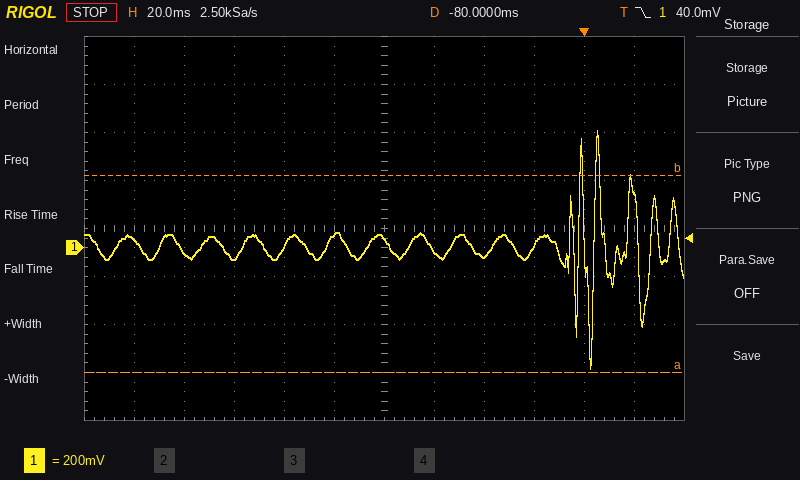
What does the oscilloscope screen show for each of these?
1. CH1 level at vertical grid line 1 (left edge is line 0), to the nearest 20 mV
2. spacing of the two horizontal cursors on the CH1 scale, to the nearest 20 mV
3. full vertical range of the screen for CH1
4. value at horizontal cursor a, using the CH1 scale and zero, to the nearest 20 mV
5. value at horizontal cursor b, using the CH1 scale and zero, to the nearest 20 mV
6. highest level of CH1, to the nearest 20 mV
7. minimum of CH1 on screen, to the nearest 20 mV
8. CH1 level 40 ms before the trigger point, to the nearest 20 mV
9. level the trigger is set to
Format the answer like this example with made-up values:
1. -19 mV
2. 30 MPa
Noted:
1. 40 mV
2. 820 mV
3. 1.6 V
4. -520 mV
5. 300 mV
6. 480 mV
7. -500 mV
8. -40 mV
9. 40.0 mV
